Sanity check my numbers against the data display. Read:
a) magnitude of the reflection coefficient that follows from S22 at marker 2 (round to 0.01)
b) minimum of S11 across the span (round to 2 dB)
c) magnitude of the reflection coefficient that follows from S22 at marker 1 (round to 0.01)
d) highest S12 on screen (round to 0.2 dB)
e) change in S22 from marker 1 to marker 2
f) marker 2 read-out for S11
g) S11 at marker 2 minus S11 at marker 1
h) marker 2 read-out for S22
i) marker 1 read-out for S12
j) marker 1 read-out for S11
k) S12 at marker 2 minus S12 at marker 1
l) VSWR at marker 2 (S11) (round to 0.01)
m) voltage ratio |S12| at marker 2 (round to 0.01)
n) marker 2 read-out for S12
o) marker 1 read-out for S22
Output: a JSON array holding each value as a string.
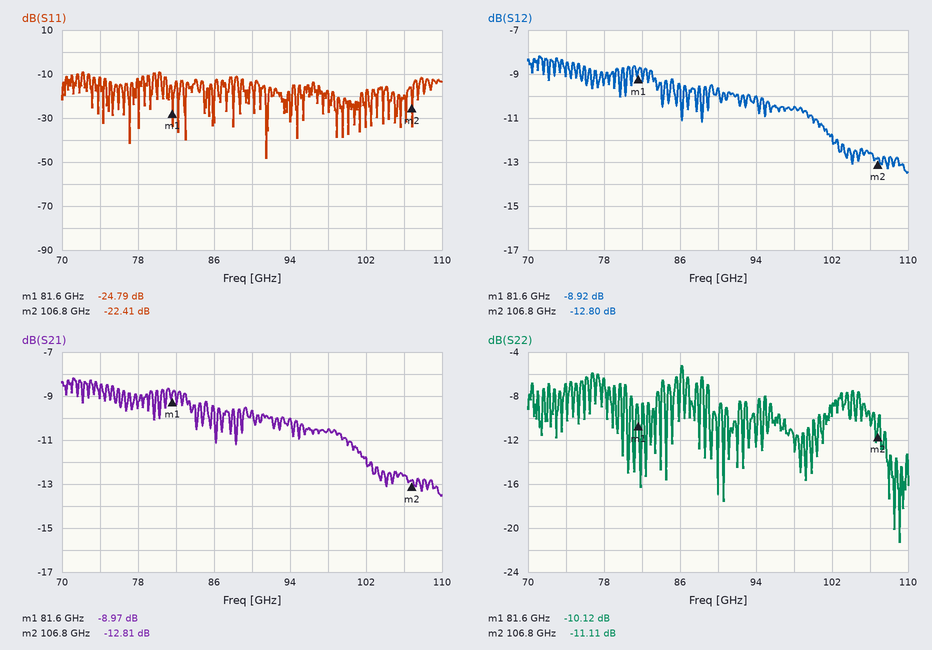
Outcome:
["0.28", "-48 dB", "0.31", "-8.2 dB", "-0.99 dB", "-22.41 dB", "2.38 dB", "-11.11 dB", "-8.92 dB", "-24.79 dB", "-3.88 dB", "1.16", "0.23", "-12.80 dB", "-10.12 dB"]
